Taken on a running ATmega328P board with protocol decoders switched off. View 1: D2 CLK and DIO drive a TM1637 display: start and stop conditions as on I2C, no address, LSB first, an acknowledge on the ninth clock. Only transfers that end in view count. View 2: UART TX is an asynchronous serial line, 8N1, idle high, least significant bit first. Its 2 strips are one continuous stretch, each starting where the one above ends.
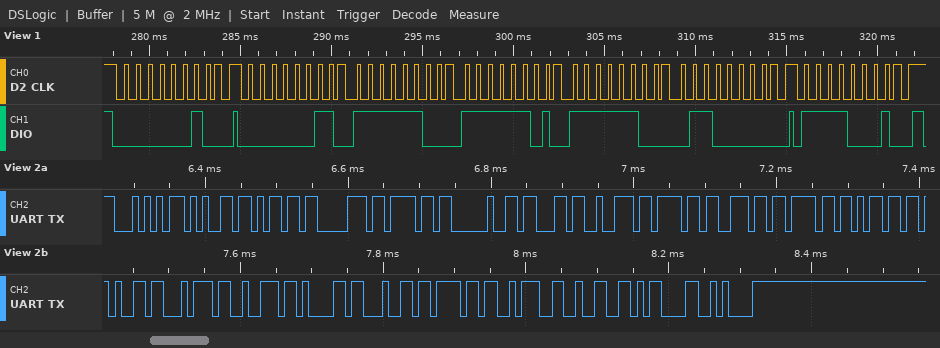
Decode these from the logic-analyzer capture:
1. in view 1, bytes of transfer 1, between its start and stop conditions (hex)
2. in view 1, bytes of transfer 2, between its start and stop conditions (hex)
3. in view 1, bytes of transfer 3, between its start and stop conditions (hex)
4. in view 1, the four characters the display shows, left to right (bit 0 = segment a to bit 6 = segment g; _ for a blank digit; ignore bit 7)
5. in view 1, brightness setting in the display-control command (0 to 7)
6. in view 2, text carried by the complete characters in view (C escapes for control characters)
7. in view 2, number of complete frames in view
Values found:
40
C0 3F BF 3F 06
8F
0001
7
"Tempo cronometrado:2\r\n"
22
